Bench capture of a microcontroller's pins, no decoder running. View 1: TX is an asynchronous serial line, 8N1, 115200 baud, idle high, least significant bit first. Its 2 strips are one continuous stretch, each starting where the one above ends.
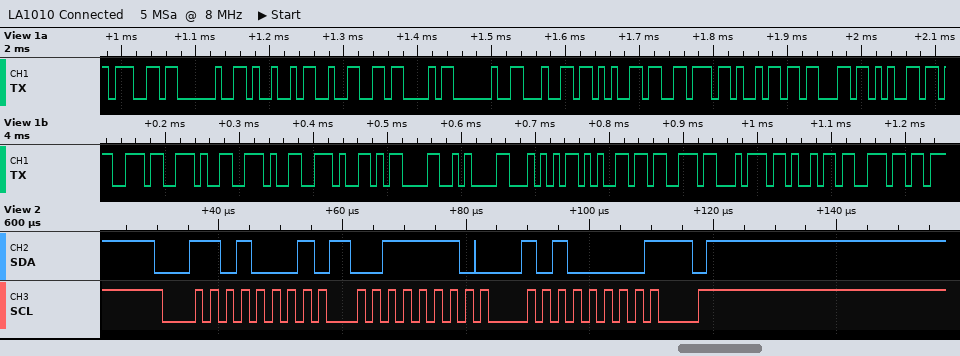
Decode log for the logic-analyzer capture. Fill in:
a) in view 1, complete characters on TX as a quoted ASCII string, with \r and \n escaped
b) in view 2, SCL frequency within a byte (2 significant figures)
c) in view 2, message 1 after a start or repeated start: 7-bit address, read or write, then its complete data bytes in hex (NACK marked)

"g I2C devices...\r\nTestin"
400 kHz
0x68 read: 3E A0 NACK
